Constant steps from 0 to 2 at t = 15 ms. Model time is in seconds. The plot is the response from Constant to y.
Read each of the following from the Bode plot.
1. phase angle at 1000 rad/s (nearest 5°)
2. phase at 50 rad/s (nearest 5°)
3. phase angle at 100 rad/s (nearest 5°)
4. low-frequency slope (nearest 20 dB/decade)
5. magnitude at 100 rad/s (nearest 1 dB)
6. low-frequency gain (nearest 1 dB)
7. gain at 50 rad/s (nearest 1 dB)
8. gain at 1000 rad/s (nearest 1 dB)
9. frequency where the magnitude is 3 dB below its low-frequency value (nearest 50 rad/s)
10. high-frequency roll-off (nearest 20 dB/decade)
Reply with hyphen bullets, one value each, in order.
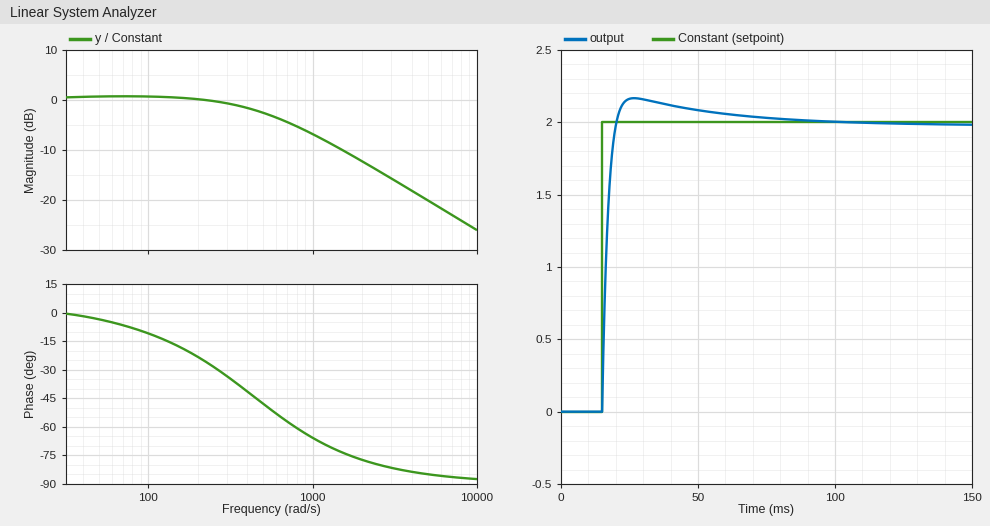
- -65°
- -5°
- -10°
- 0 dB/decade
- 1 dB
- 1 dB
- 1 dB
- -7 dB
- 500 rad/s
- -20 dB/decade
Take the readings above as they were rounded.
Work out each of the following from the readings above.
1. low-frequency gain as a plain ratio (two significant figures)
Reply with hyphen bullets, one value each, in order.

- 1.1
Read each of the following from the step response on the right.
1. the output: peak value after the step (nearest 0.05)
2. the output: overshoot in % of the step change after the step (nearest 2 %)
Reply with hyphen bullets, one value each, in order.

- 2.15
- 10 %
